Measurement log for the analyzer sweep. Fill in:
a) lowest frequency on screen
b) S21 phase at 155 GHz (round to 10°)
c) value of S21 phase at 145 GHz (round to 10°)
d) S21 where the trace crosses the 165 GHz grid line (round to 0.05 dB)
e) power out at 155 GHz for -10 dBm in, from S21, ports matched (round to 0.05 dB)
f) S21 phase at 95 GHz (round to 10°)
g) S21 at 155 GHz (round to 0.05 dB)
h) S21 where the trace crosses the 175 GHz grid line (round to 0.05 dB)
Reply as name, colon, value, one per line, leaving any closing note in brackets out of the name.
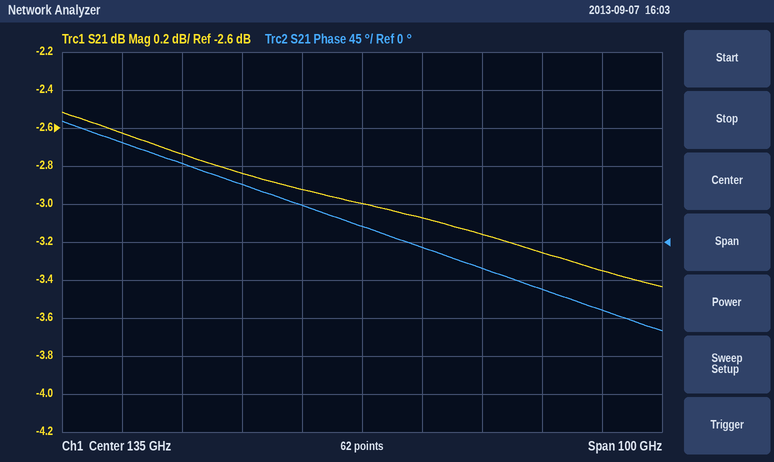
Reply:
lowest frequency on screen: 85 GHz
S21 phase at 155 GHz: -30°
value of S21 phase at 145 GHz: -10°
S21 where the trace crosses the 165 GHz grid line: -3.25 dB
power out at 155 GHz for -10 dBm in, from S21, ports matched: -13.15 dBm
S21 phase at 95 GHz: 120°
S21 at 155 GHz: -3.15 dB
S21 where the trace crosses the 175 GHz grid line: -3.35 dB
